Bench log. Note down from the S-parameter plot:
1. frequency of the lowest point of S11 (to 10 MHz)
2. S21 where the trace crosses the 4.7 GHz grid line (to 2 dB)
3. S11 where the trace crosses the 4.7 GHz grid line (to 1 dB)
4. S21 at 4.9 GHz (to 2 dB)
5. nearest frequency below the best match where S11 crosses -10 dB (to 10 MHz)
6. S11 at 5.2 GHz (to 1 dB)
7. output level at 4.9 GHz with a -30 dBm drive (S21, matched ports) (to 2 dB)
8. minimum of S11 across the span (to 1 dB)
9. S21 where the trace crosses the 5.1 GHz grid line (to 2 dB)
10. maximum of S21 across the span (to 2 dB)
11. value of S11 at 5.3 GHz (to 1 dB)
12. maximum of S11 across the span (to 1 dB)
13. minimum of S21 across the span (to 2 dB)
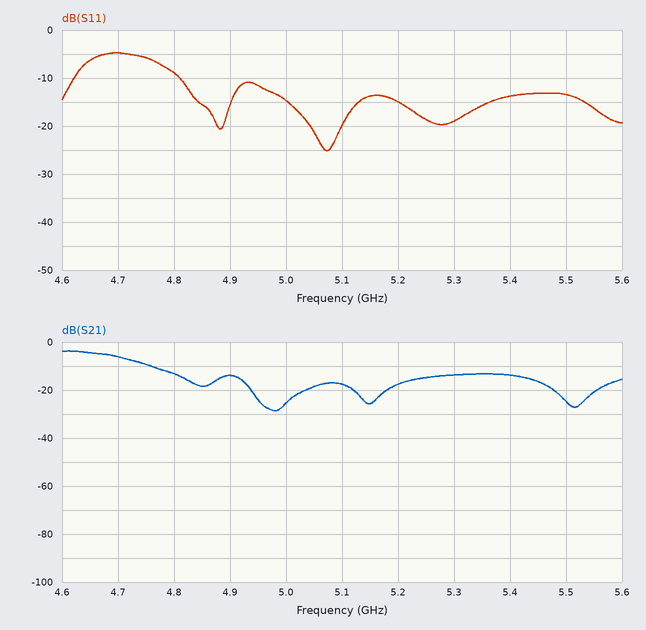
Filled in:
5.07 GHz
-6 dB
-5 dB
-14 dB
4.81 GHz
-15 dB
-44 dBm
-25 dB
-18 dB
-4 dB
-19 dB
-5 dB
-28 dB
